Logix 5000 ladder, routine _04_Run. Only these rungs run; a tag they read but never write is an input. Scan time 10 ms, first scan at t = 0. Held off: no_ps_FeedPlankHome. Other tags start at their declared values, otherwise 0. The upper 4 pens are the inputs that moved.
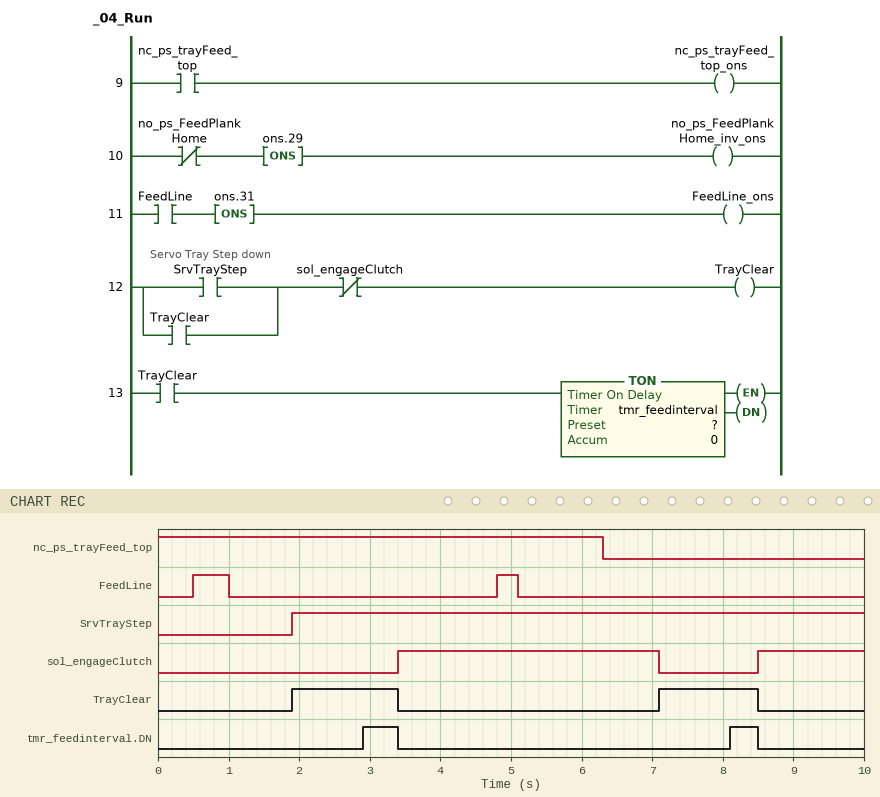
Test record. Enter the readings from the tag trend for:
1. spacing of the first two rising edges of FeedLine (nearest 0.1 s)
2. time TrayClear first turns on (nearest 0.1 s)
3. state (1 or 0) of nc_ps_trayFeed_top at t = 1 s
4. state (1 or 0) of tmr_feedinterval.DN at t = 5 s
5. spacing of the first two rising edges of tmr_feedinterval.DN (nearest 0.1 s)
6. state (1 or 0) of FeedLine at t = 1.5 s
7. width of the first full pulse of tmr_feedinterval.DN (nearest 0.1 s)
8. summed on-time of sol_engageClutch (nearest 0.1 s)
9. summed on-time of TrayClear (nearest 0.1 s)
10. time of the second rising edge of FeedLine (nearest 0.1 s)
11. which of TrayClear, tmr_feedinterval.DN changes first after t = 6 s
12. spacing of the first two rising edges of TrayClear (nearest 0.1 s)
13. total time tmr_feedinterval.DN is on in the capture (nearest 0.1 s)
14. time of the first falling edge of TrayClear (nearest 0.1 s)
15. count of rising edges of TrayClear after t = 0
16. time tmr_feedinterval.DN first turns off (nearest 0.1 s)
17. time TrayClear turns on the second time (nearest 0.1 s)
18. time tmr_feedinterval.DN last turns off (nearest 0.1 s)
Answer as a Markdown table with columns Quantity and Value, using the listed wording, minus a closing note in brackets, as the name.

| Quantity | Value |
|---|---|
| spacing of the first two rising edges of FeedLine | 4.3 s |
| time TrayClear first turns on | 1.9 s |
| state (1 or 0) of nc_ps_trayFeed_top at t = 1 s | 1 |
| state (1 or 0) of tmr_feedinterval.DN at t = 5 s | 0 |
| spacing of the first two rising edges of tmr_feedinterval.DN | 5.2 s |
| state (1 or 0) of FeedLine at t = 1.5 s | 0 |
| width of the first full pulse of tmr_feedinterval.DN | 0.5 s |
| summed on-time of sol_engageClutch | 5.2 s |
| summed on-time of TrayClear | 2.9 s |
| time of the second rising edge of FeedLine | 4.8 s |
| which of TrayClear, tmr_feedinterval.DN changes first after t = 6 s | TrayClear |
| spacing of the first two rising edges of TrayClear | 5.2 s |
| total time tmr_feedinterval.DN is on in the capture | 0.9 s |
| time of the first falling edge of TrayClear | 3.4 s |
| count of rising edges of TrayClear after t = 0 | 2 |
| time tmr_feedinterval.DN first turns off | 3.4 s |
| time TrayClear turns on the second time | 7.1 s |
| time tmr_feedinterval.DN last turns off | 8.5 s |
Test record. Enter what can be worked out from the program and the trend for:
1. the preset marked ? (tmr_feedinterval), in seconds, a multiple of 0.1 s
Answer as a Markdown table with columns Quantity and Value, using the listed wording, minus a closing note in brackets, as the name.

| Quantity | Value |
|---|---|
| the preset marked ? (tmr_feedinterval), in seconds, a multiple of 0.1 s | 1.0 s |
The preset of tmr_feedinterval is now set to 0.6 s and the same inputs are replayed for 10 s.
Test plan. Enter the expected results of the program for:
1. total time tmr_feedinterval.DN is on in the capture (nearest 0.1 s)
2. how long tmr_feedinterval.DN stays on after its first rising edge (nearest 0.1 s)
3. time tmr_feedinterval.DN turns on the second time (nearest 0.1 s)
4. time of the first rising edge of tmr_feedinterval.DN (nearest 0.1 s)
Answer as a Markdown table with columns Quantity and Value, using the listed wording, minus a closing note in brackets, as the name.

| Quantity | Value |
|---|---|
| total time tmr_feedinterval.DN is on in the capture | 1.7 s |
| how long tmr_feedinterval.DN stays on after its first rising edge | 0.9 s |
| time tmr_feedinterval.DN turns on the second time | 7.7 s |
| time of the first rising edge of tmr_feedinterval.DN | 2.5 s |
